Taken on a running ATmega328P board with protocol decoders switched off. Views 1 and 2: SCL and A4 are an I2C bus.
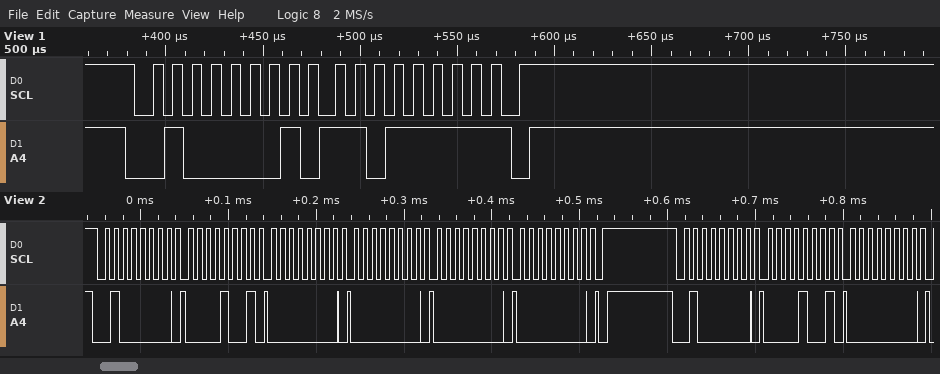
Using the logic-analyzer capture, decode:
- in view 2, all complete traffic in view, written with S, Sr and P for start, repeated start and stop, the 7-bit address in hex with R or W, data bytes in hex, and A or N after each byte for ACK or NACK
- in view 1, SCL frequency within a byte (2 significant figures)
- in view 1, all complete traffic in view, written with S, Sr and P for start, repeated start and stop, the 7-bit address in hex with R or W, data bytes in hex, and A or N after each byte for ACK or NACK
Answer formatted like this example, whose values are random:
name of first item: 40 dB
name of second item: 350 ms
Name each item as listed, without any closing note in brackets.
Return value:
in view 2, all complete traffic in view, written with S, Sr and P for start, repeated start and stop, the 7-bit address in hex with R or W, data bytes in hex, and A or N after each byte for ACK or NACK: S 20W A 09 A 00 A 00 A 00 A 00 A P S 20W A 09 A 00 A
in view 1, SCL frequency within a byte: 100 kHz
in view 1, all complete traffic in view, written with S, Sr and P for start, repeated start and stop, the 7-bit address in hex with R or W, data bytes in hex, and A or N after each byte for ACK or NACK: S 20R A DF N P
